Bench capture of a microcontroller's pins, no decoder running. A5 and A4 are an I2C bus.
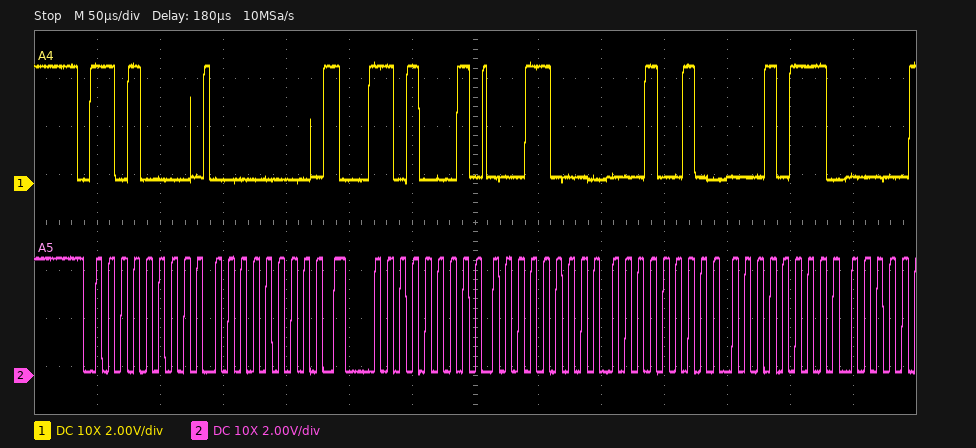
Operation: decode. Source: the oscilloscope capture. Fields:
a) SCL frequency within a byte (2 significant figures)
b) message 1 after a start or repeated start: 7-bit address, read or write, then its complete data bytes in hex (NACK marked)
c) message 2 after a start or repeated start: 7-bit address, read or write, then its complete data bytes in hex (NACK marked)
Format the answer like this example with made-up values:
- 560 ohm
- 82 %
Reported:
- 100 kHz
- 0x68 write: 00
- 0x68 read: 18 12 17
